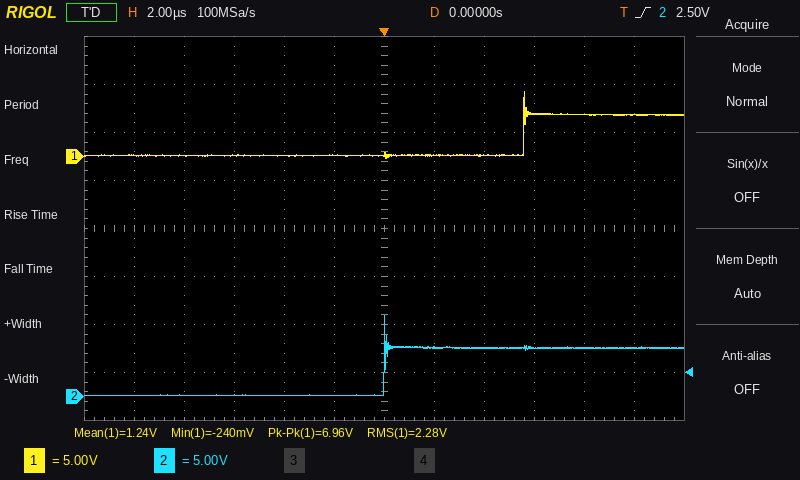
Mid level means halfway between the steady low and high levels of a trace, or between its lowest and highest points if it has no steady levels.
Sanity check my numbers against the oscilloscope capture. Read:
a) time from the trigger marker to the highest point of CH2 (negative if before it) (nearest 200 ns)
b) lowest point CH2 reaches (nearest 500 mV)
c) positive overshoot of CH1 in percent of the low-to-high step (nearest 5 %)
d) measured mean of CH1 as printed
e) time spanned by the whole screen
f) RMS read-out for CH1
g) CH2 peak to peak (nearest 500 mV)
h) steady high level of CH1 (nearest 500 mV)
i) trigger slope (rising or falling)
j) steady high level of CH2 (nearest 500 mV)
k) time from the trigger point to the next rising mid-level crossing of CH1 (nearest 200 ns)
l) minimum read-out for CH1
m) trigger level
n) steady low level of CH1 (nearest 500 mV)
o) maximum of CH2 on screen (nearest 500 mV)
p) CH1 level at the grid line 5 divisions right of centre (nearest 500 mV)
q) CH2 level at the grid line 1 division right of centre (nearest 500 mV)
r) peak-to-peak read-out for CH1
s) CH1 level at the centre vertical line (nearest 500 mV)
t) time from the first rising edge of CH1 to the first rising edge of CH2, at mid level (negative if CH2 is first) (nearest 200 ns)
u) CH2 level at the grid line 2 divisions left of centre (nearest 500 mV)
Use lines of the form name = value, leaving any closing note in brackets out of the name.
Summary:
time from the trigger marker to the highest point of CH2 (negative if before it) = 0.0 µs
lowest point CH2 reaches = 0.0 V
positive overshoot of CH1 in percent of the low-to-high step = 55 %
measured mean of CH1 as printed = 1.24 V
time spanned by the whole screen = 24 µs
RMS read-out for CH1 = 2.28 V
CH2 peak to peak = 8.5 V
steady high level of CH1 = 4.5 V
trigger slope = rising
steady high level of CH2 = 5.0 V
time from the trigger point to the next rising mid-level crossing of CH1 = 5.6 µs
minimum read-out for CH1 = -240 mV
trigger level = 2.50 V
steady low level of CH1 = 0.0 V
maximum of CH2 on screen = 8.5 V
CH1 level at the grid line 5 divisions right of centre = 4.5 V
CH2 level at the grid line 1 division right of centre = 5.0 V
peak-to-peak read-out for CH1 = 6.96 V
CH1 level at the centre vertical line = 0.0 V
time from the first rising edge of CH1 to the first rising edge of CH2, at mid level (negative if CH2 is first) = -5.6 µs
CH2 level at the grid line 2 divisions left of centre = 0.0 V
